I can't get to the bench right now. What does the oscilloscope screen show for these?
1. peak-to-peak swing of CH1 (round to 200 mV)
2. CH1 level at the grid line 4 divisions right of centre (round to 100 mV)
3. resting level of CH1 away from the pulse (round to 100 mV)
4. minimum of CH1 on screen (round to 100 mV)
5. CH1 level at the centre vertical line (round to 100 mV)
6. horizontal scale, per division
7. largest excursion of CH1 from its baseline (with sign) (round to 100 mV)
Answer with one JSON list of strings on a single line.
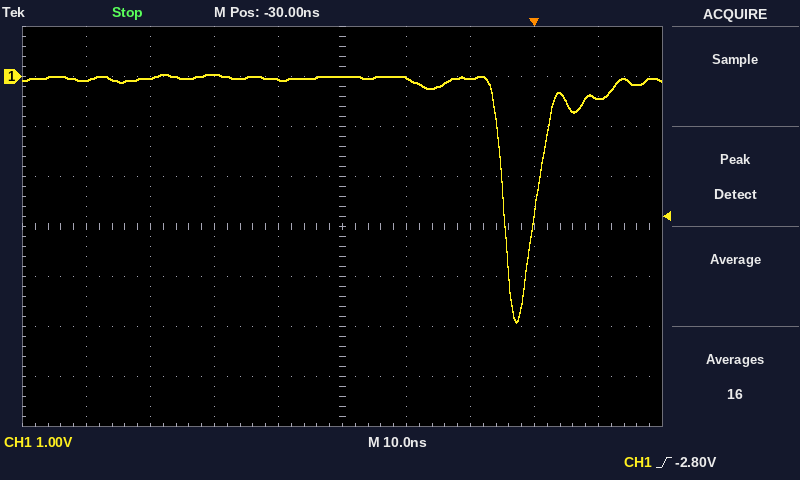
["5.0 V", "-400 mV", "0.0 V", "-4.9 V", "0.0 V", "10 ns", "-4.9 V"]
